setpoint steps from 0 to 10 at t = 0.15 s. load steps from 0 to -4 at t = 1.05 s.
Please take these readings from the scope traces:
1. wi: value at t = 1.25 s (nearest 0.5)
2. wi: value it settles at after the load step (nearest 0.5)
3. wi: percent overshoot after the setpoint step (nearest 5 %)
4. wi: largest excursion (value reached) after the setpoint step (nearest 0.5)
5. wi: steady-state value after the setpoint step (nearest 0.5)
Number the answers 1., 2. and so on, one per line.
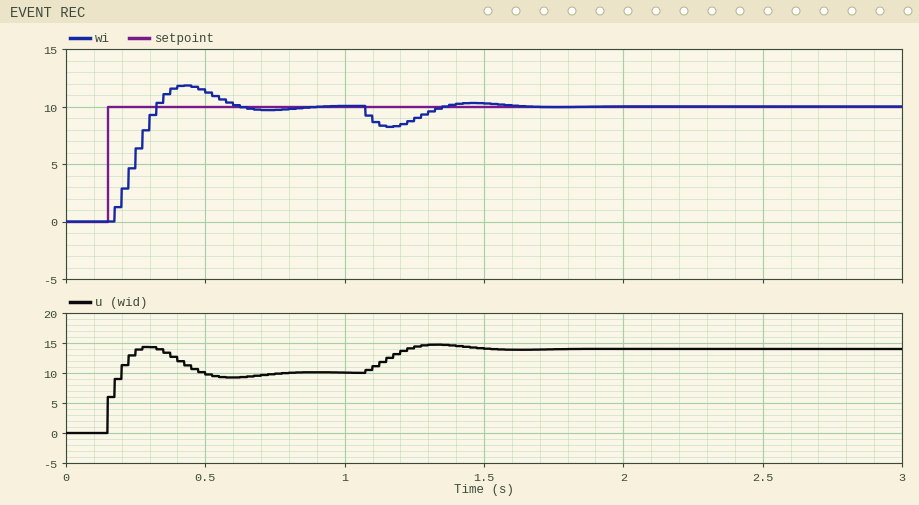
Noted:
1. 9.0
2. 10.0
3. 20 %
4. 12.0
5. 10.0
